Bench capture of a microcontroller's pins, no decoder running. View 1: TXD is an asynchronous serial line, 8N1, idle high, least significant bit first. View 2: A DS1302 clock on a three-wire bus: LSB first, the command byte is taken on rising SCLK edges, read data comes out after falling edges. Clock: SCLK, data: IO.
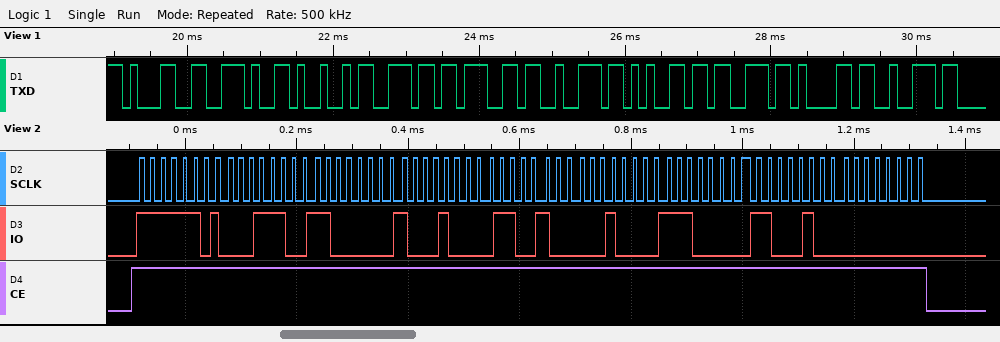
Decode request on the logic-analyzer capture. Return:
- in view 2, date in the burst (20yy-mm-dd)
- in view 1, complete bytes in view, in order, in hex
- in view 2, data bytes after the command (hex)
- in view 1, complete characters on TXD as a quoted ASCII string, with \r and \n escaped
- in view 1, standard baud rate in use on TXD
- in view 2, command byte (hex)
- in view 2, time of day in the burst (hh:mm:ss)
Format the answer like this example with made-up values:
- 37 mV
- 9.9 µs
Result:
- 2023-08-26
- 31 2E 49 6E 67 72 65 73 61 72
- 38 03 11 26 08 07 23 00
- "1.Ingresar"
- 9600 baud
- 0xBF
- 11:03:38
